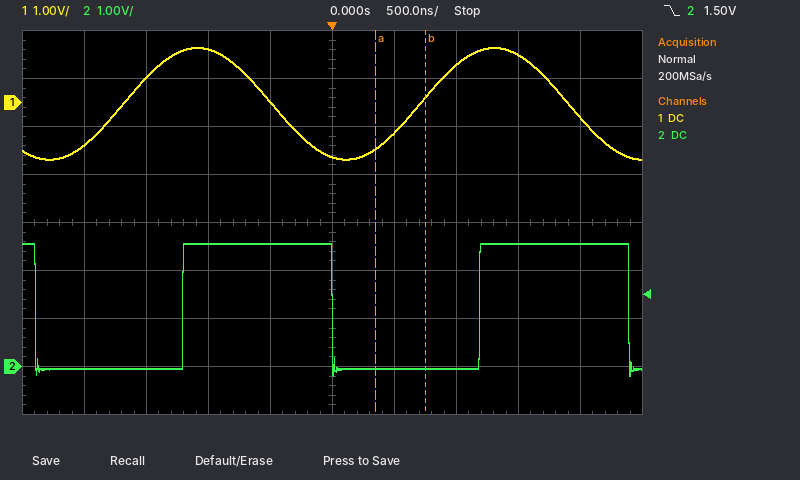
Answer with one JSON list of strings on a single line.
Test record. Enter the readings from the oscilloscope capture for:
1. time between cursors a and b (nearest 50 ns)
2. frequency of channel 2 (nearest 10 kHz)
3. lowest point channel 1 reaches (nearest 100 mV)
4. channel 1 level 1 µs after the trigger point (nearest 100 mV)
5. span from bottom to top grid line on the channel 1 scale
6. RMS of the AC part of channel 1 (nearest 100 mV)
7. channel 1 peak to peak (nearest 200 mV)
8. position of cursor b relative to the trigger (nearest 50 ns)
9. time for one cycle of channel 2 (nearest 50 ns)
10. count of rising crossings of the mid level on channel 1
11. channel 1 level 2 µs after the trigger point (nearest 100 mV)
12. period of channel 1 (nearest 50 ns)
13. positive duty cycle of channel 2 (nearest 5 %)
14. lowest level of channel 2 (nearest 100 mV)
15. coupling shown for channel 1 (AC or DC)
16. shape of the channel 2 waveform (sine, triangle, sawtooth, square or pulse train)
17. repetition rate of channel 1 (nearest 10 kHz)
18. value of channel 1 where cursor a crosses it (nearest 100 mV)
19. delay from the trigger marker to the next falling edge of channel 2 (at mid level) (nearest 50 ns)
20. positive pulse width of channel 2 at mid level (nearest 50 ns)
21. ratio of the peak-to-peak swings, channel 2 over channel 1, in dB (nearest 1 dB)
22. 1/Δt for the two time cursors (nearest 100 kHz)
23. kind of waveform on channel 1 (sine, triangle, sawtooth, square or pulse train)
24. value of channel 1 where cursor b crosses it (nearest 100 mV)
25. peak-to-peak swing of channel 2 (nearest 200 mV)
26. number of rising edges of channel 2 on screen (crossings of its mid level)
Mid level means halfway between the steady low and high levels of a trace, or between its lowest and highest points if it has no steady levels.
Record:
["400 ns", "420 kHz", "-1.2 V", "800 mV", "8 V", "800 mV", "2.4 V", "+750 ns", "2.40 µs", "2", "-300 mV", "2.40 µs", "50 %", "-200 mV", "DC", "square", "420 kHz", "-1.0 V", "2.40 µs", "1.20 µs", "1 dB", "2.5 MHz", "sine", "100 mV", "2.8 V", "2"]
